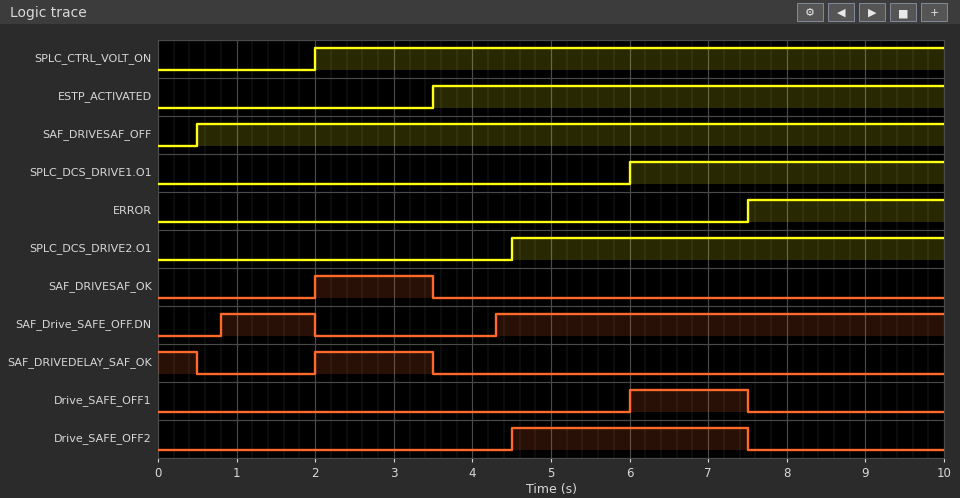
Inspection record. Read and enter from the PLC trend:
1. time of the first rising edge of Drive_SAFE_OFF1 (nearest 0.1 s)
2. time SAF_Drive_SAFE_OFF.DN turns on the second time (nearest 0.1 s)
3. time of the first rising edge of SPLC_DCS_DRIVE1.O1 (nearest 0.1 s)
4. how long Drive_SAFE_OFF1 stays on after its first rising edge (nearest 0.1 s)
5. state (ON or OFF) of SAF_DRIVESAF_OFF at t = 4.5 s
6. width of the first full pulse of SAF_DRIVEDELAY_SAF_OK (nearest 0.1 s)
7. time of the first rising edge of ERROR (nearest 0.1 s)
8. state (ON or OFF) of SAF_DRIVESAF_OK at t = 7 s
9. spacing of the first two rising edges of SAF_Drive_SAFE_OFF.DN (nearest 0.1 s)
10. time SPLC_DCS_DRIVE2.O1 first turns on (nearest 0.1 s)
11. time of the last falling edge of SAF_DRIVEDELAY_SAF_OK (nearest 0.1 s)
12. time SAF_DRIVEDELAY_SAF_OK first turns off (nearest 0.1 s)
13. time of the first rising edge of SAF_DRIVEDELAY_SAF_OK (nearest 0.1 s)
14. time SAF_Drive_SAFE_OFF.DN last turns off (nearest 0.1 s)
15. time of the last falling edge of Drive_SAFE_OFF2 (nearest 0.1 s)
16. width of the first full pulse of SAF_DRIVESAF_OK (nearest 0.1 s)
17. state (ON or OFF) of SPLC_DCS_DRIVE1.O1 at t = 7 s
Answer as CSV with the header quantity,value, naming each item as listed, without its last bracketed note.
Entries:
quantity,value
time of the first rising edge of Drive_SAFE_OFF1,6.0 s
time SAF_Drive_SAFE_OFF.DN turns on the second time,4.3 s
time of the first rising edge of SPLC_DCS_DRIVE1.O1,6.0 s
how long Drive_SAFE_OFF1 stays on after its first rising edge,1.5 s
state (ON or OFF) of SAF_DRIVESAF_OFF at t = 4.5 s,ON
width of the first full pulse of SAF_DRIVEDELAY_SAF_OK,1.5 s
time of the first rising edge of ERROR,7.5 s
state (ON or OFF) of SAF_DRIVESAF_OK at t = 7 s,OFF
spacing of the first two rising edges of SAF_Drive_SAFE_OFF.DN,3.5 s
time SPLC_DCS_DRIVE2.O1 first turns on,4.5 s
time of the last falling edge of SAF_DRIVEDELAY_SAF_OK,3.5 s
time SAF_DRIVEDELAY_SAF_OK first turns off,0.5 s
time of the first rising edge of SAF_DRIVEDELAY_SAF_OK,2.0 s
time SAF_Drive_SAFE_OFF.DN last turns off,2.0 s
time of the last falling edge of Drive_SAFE_OFF2,7.5 s
width of the first full pulse of SAF_DRIVESAF_OK,1.5 s
state (ON or OFF) of SPLC_DCS_DRIVE1.O1 at t = 7 s,ON
